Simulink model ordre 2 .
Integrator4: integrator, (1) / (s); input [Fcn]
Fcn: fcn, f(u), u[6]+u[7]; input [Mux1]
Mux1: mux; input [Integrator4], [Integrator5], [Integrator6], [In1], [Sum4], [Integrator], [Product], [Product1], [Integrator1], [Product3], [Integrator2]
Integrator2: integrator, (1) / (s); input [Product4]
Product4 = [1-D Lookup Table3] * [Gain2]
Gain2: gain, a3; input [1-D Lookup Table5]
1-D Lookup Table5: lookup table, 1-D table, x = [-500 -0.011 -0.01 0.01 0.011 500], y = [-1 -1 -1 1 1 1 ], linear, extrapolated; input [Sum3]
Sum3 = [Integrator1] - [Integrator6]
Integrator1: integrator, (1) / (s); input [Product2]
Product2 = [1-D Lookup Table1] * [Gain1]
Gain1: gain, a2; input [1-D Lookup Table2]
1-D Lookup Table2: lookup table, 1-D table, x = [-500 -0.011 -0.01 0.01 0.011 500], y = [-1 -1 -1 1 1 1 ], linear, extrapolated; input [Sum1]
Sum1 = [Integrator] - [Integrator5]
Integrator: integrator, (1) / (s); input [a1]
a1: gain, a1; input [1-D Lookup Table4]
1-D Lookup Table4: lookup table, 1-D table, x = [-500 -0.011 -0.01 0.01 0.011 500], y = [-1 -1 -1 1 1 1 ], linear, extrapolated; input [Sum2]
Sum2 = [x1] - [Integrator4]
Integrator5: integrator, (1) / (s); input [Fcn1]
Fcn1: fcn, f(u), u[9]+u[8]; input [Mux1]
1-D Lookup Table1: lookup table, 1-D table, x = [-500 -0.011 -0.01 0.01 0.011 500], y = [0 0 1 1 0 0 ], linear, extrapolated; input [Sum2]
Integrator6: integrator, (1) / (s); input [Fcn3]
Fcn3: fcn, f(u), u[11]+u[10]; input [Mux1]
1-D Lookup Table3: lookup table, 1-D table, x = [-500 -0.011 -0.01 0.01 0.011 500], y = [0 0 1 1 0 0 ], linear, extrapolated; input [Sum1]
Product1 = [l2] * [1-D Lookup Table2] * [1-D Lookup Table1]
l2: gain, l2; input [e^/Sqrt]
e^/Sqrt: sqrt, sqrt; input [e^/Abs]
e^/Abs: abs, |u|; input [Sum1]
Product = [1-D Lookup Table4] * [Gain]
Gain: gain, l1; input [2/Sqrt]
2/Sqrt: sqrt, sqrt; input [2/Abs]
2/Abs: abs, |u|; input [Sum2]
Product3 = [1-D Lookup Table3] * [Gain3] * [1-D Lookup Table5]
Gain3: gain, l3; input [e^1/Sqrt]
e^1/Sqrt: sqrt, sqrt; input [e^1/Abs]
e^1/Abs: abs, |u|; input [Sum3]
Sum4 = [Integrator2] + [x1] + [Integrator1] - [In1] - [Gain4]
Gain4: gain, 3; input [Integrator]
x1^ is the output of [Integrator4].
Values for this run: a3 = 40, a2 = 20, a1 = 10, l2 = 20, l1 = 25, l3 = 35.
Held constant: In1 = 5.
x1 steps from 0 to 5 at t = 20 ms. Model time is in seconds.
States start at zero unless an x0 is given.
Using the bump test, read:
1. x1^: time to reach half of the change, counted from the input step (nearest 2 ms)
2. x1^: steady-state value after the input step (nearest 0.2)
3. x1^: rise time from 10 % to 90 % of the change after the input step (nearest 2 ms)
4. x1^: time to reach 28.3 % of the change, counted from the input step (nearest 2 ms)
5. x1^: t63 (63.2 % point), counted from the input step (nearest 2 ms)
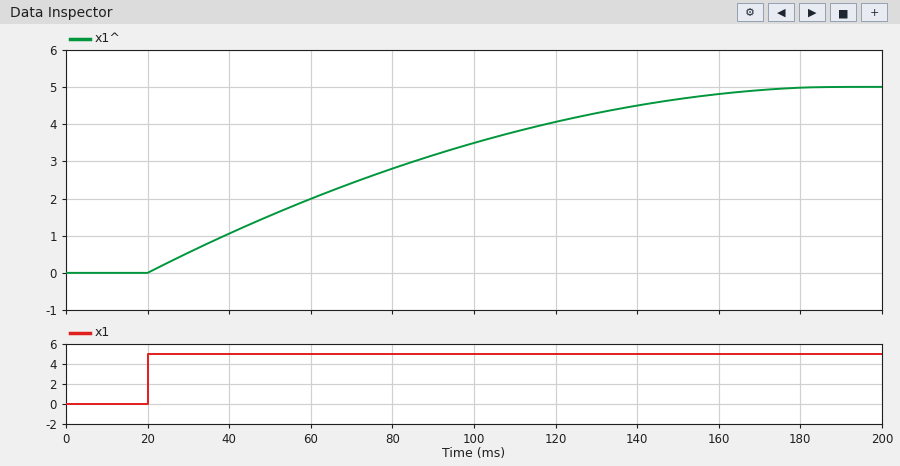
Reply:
52 ms
5.0
110 ms
28 ms
70 ms
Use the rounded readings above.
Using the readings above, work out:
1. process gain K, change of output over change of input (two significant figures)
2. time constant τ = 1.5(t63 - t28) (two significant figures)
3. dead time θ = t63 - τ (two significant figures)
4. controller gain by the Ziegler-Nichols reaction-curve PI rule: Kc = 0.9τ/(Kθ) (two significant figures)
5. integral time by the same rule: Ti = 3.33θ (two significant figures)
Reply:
1.0
63 ms
7.0 ms
8.1
23 ms
